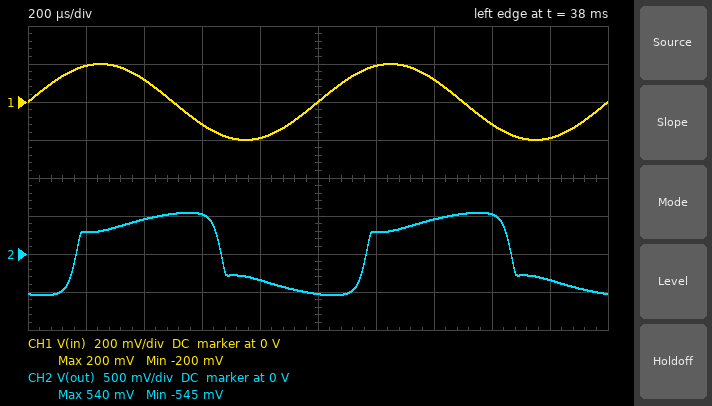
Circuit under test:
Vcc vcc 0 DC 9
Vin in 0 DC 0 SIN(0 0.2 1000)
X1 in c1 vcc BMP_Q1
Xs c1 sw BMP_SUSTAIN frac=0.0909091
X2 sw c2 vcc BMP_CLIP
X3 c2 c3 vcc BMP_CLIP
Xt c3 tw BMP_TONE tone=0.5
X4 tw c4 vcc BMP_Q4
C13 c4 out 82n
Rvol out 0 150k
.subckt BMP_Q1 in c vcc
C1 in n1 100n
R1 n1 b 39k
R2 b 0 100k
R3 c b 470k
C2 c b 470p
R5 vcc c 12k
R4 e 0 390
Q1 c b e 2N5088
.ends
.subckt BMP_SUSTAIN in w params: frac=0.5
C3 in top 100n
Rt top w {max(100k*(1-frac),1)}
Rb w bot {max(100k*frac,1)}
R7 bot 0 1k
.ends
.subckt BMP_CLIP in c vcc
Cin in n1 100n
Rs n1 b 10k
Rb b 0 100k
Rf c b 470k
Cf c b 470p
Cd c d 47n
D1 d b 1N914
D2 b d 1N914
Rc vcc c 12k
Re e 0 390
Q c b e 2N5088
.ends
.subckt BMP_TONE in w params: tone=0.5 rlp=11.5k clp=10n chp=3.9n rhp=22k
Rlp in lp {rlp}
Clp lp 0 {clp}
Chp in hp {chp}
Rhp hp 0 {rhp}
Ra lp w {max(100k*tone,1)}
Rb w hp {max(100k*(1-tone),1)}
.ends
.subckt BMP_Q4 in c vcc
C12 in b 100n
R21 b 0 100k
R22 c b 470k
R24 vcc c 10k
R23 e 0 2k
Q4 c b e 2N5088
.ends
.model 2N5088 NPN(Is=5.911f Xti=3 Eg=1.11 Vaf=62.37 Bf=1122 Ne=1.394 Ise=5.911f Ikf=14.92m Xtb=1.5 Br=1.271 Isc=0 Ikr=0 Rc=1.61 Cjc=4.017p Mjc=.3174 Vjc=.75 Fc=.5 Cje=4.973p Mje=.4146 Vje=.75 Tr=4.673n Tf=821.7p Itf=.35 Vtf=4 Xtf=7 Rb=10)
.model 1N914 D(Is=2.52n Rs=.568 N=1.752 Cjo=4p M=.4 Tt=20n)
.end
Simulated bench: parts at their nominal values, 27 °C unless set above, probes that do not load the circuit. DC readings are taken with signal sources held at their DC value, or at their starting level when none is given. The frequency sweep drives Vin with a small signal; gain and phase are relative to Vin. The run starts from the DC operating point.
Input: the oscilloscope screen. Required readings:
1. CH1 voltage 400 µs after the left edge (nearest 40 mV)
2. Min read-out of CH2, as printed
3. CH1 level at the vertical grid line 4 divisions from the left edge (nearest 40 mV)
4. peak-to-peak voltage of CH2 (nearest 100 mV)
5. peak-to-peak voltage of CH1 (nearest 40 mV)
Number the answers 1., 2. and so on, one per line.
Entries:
1. 120 mV
2. -545 mV
3. -200 mV
4. 1.1 V
5. 400 mV
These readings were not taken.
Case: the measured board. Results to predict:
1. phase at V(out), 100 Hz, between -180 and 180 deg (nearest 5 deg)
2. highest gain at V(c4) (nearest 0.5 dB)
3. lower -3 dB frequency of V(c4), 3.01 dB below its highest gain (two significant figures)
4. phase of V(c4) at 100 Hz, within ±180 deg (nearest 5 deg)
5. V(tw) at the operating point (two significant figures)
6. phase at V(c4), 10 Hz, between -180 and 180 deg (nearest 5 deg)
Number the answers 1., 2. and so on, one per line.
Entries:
1. 80 deg
2. 38.0 dB
3. 71 Hz
4. 70 deg
5. 2.5 V
6. -15 deg
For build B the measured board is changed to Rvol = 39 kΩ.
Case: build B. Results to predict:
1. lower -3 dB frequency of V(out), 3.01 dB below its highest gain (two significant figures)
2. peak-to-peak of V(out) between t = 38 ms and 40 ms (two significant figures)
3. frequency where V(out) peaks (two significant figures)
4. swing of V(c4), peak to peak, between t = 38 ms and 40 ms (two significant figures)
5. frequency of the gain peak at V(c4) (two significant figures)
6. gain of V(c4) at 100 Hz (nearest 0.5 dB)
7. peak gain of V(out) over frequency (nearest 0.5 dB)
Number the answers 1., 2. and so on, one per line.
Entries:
1. 81 Hz
2. 930 mV
3. 220 Hz
4. 960 mV
5. 200 Hz
6. 36.0 dB
7. 37.0 dB
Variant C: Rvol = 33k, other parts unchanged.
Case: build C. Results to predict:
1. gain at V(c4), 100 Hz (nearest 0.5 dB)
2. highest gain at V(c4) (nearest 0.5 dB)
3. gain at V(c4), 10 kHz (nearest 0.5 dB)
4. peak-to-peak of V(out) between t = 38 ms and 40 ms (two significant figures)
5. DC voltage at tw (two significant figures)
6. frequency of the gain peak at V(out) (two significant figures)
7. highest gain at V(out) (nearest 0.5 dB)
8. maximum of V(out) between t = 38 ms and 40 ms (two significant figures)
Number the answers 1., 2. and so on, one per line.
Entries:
1. 36.0 dB
2. 37.0 dB
3. -9.0 dB
4. 900 mV
5. 2.5 V
6. 230 Hz
7. 36.5 dB
8. 450 mV
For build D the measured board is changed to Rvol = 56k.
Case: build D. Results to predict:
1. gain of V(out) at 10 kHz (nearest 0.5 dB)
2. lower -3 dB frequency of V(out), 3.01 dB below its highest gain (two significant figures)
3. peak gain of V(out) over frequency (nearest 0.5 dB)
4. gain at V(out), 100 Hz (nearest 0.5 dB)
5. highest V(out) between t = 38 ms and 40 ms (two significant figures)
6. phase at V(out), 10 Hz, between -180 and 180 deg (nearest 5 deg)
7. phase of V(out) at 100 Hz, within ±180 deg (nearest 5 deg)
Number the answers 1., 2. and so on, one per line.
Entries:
1. -8.5 dB
2. 77 Hz
3. 37.5 dB
4. 36.0 dB
5. 490 mV
6. 60 deg
7. 90 deg
